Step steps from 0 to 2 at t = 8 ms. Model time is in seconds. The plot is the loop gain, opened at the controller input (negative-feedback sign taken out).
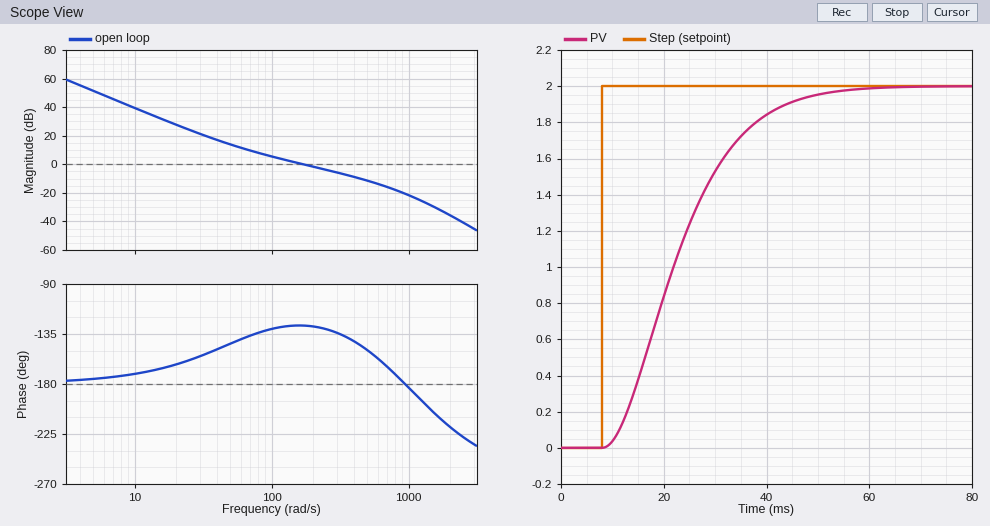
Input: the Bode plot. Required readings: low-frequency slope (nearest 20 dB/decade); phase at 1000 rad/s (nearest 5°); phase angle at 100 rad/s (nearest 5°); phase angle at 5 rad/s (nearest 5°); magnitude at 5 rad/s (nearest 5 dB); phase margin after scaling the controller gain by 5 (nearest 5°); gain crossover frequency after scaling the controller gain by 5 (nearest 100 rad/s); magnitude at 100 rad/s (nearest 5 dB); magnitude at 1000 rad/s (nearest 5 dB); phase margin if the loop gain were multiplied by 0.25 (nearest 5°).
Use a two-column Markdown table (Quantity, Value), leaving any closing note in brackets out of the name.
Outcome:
| Quantity | Value |
|---|---|
| low-frequency slope | -40 dB/decade |
| phase at 1000 rad/s | -185° |
| phase angle at 100 rad/s | -130° |
| phase angle at 5 rad/s | -175° |
| magnitude at 5 rad/s | 50 dB |
| phase margin after scaling the controller gain by 5 | 20° |
| gain crossover frequency after scaling the controller gain by 5 | 600 rad/s |
| magnitude at 100 rad/s | 5 dB |
| magnitude at 1000 rad/s | -20 dB |
| phase margin if the loop gain were multiplied by 0.25 | 40° |
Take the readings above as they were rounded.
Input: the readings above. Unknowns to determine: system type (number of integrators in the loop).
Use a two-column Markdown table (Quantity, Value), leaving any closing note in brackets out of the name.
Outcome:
| Quantity | Value |
|---|---|
| system type | 2 |
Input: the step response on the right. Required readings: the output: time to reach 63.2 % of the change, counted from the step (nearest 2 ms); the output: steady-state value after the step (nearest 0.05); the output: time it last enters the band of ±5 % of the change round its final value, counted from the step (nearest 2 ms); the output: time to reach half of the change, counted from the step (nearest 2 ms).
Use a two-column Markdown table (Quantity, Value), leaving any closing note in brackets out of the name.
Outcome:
| Quantity | Value |
|---|---|
| the output: time to reach 63.2 % of the change, counted from the step | 18 ms |
| the output: steady-state value after the step | 2.00 |
| the output: time it last enters the band of ±5 % of the change round its final value, counted from the step | 36 ms |
| the output: time to reach half of the change, counted from the step | 14 ms |
